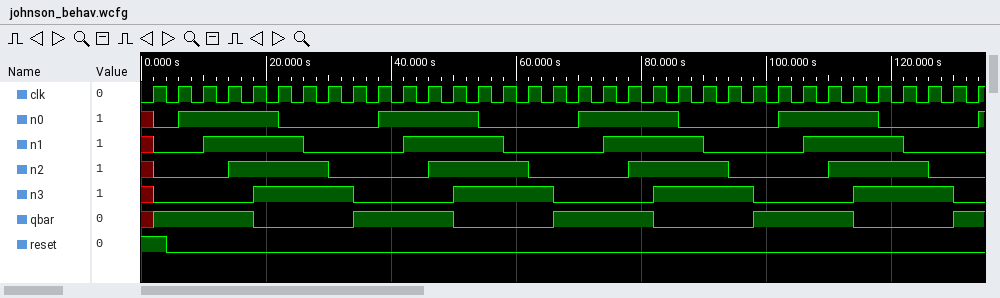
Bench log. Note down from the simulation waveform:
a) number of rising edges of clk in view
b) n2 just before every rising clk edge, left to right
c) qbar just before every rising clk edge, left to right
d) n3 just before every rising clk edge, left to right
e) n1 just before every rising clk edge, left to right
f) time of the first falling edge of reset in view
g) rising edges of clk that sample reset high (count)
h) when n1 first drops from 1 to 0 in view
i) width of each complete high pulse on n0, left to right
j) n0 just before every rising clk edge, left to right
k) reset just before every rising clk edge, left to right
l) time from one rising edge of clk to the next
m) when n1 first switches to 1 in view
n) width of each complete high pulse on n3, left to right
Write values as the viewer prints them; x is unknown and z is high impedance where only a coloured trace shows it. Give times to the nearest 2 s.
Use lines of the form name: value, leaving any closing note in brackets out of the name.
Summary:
number of rising edges of clk in view: 34
n2 just before every rising clk edge, left to right: x 0 0 0 1 1 1 1 0 0 0 0 1 1 1 1 0 0 0 0 1 1 1 1 0 0 0 0 1 1 1 1 0 0
qbar just before every rising clk edge, left to right: x 1 1 1 1 0 0 0 0 1 1 1 1 0 0 0 0 1 1 1 1 0 0 0 0 1 1 1 1 0 0 0 0 1
n3 just before every rising clk edge, left to right: x 0 0 0 0 1 1 1 1 0 0 0 0 1 1 1 1 0 0 0 0 1 1 1 1 0 0 0 0 1 1 1 1 0
n1 just before every rising clk edge, left to right: x 0 0 1 1 1 1 0 0 0 0 1 1 1 1 0 0 0 0 1 1 1 1 0 0 0 0 1 1 1 1 0 0 0
time of the first falling edge of reset in view: 4 s
rising edges of clk that sample reset high: 1
when n1 first drops from 1 to 0 in view: 26 s
width of each complete high pulse on n0, left to right: 16 s, 16 s, 16 s, 16 s
n0 just before every rising clk edge, left to right: x 0 1 1 1 1 0 0 0 0 1 1 1 1 0 0 0 0 1 1 1 1 0 0 0 0 1 1 1 1 0 0 0 0
reset just before every rising clk edge, left to right: 1 0 0 0 0 0 0 0 0 0 0 0 0 0 0 0 0 0 0 0 0 0 0 0 0 0 0 0 0 0 0 0 0 0
time from one rising edge of clk to the next: 4 s
when n1 first switches to 1 in view: 10 s
width of each complete high pulse on n3, left to right: 16 s, 16 s, 16 s, 16 s
